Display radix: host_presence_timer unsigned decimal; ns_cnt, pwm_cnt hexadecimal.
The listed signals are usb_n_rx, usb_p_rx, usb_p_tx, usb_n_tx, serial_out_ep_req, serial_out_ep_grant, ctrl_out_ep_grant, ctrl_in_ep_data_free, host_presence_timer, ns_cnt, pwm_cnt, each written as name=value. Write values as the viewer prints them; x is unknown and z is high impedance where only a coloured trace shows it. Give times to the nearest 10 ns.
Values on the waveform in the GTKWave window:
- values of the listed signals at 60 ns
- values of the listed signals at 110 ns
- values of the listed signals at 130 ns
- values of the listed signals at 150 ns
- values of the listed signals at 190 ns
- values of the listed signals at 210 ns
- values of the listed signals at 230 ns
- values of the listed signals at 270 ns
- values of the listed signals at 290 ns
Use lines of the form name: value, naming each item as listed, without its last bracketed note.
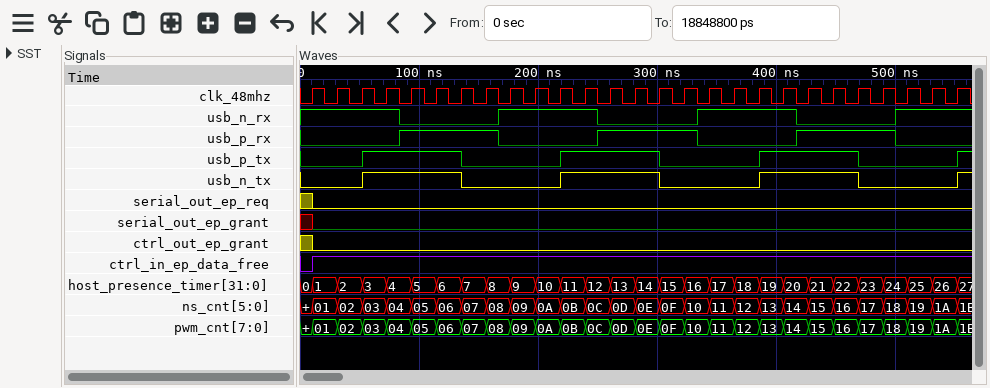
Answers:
values of the listed signals at 60 ns: usb_n_rx=1, usb_p_rx=0, usb_p_tx=1, usb_n_tx=1, serial_out_ep_req=0, serial_out_ep_grant=0, ctrl_out_ep_grant=0, ctrl_in_ep_data_free=1, host_presence_timer=3, ns_cnt=03, pwm_cnt=03
values of the listed signals at 110 ns: usb_n_rx=0, usb_p_rx=1, usb_p_tx=1, usb_n_tx=1, serial_out_ep_req=0, serial_out_ep_grant=0, ctrl_out_ep_grant=0, ctrl_in_ep_data_free=1, host_presence_timer=5, ns_cnt=05, pwm_cnt=05
values of the listed signals at 130 ns: usb_n_rx=0, usb_p_rx=1, usb_p_tx=1, usb_n_tx=1, serial_out_ep_req=0, serial_out_ep_grant=0, ctrl_out_ep_grant=0, ctrl_in_ep_data_free=1, host_presence_timer=6, ns_cnt=06, pwm_cnt=06
values of the listed signals at 150 ns: usb_n_rx=0, usb_p_rx=1, usb_p_tx=0, usb_n_tx=0, serial_out_ep_req=0, serial_out_ep_grant=0, ctrl_out_ep_grant=0, ctrl_in_ep_data_free=1, host_presence_timer=7, ns_cnt=07, pwm_cnt=07
values of the listed signals at 190 ns: usb_n_rx=1, usb_p_rx=0, usb_p_tx=0, usb_n_tx=0, serial_out_ep_req=0, serial_out_ep_grant=0, ctrl_out_ep_grant=0, ctrl_in_ep_data_free=1, host_presence_timer=9, ns_cnt=09, pwm_cnt=09
values of the listed signals at 210 ns: usb_n_rx=1, usb_p_rx=0, usb_p_tx=0, usb_n_tx=0, serial_out_ep_req=0, serial_out_ep_grant=0, ctrl_out_ep_grant=0, ctrl_in_ep_data_free=1, host_presence_timer=10, ns_cnt=0A, pwm_cnt=0A
values of the listed signals at 230 ns: usb_n_rx=1, usb_p_rx=0, usb_p_tx=1, usb_n_tx=1, serial_out_ep_req=0, serial_out_ep_grant=0, ctrl_out_ep_grant=0, ctrl_in_ep_data_free=1, host_presence_timer=11, ns_cnt=0B, pwm_cnt=0B
values of the listed signals at 270 ns: usb_n_rx=0, usb_p_rx=1, usb_p_tx=1, usb_n_tx=1, serial_out_ep_req=0, serial_out_ep_grant=0, ctrl_out_ep_grant=0, ctrl_in_ep_data_free=1, host_presence_timer=13, ns_cnt=0D, pwm_cnt=0D
values of the listed signals at 290 ns: usb_n_rx=0, usb_p_rx=1, usb_p_tx=1, usb_n_tx=1, serial_out_ep_req=0, serial_out_ep_grant=0, ctrl_out_ep_grant=0, ctrl_in_ep_data_free=1, host_presence_timer=14, ns_cnt=0E, pwm_cnt=0E
